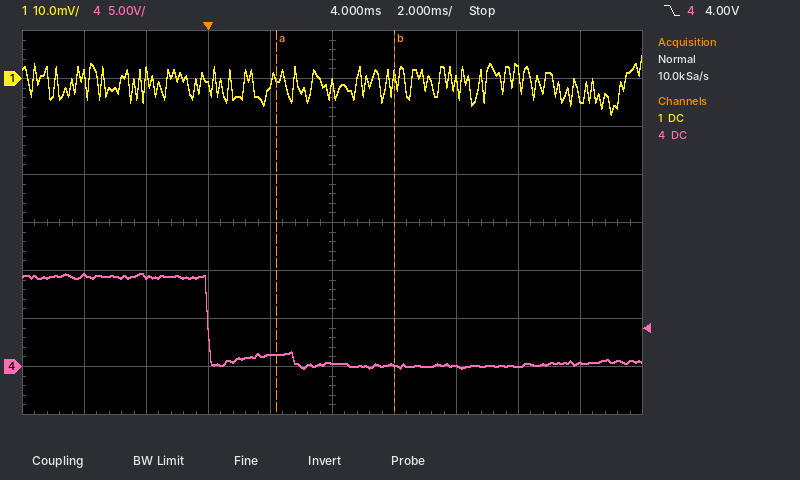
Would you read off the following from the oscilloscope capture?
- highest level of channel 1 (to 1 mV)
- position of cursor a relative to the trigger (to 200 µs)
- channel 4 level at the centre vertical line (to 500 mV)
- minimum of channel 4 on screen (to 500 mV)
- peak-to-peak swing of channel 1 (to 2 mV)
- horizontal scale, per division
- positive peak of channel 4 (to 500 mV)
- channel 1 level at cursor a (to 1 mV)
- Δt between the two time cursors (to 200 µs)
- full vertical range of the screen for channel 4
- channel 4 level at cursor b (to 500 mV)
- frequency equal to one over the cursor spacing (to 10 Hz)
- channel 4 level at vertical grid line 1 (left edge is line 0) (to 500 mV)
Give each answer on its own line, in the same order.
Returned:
5 mV
+2.2 ms
500 mV
0.0 V
12 mV
2 ms
9.5 V
0 mV
3.8 ms
40 V
0.0 V
260 Hz
9.5 V
